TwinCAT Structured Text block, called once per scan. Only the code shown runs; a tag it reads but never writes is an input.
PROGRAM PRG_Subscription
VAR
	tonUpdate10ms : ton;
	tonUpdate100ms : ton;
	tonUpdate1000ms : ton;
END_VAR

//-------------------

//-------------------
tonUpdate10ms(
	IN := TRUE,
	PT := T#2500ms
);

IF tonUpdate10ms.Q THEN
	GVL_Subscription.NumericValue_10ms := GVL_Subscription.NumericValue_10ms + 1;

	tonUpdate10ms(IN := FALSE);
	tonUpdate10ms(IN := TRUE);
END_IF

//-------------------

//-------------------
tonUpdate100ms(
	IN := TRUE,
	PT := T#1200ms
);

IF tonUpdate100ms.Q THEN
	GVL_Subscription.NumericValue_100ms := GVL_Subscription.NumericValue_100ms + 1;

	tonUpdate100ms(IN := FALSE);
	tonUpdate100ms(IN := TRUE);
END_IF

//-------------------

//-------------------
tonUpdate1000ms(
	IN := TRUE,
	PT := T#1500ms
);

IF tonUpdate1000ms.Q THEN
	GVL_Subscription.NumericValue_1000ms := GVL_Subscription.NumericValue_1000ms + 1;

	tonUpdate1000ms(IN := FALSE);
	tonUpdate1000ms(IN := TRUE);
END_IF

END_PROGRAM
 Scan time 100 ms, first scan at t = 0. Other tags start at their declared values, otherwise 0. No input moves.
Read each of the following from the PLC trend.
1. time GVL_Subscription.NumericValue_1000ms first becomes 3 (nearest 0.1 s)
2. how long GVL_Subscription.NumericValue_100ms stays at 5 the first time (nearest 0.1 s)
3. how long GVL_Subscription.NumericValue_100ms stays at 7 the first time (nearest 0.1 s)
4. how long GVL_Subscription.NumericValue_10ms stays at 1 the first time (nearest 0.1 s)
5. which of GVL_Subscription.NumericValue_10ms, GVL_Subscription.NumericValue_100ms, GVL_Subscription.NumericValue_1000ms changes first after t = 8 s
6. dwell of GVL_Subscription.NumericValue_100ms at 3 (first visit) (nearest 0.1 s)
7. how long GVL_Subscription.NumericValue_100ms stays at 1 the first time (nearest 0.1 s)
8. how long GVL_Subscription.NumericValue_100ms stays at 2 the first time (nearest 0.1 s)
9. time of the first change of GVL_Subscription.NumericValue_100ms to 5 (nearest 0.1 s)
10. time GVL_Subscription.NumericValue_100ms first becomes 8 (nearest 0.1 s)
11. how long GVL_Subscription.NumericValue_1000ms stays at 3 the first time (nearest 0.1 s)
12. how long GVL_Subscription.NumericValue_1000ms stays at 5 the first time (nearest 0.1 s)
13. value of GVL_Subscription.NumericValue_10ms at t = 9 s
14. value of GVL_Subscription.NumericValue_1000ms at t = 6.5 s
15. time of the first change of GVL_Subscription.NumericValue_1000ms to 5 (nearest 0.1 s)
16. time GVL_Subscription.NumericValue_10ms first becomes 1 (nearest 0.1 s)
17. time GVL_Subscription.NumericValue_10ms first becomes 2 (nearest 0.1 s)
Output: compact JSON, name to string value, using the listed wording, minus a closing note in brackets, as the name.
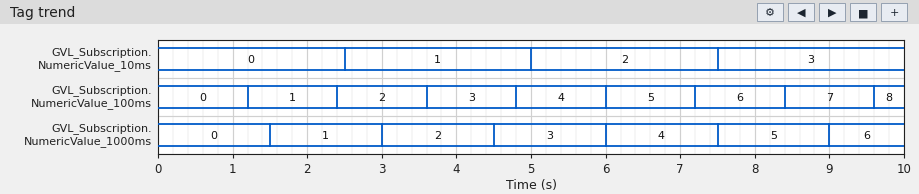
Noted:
{"time GVL_Subscription.NumericValue_1000ms first becomes 3": "4.5 s", "how long GVL_Subscription.NumericValue_100ms stays at 5 the first time": "1.2 s", "how long GVL_Subscription.NumericValue_100ms stays at 7 the first time": "1.2 s", "how long GVL_Subscription.NumericValue_10ms stays at 1 the first time": "2.5 s", "which of GVL_Subscription.NumericValue_10ms, GVL_Subscription.NumericValue_100ms, GVL_Subscription.NumericValue_1000ms changes first after t = 8 s": "GVL_Subscription.NumericValue_100ms", "dwell of GVL_Subscription.NumericValue_100ms at 3 (first visit)": "1.2 s", "how long GVL_Subscription.NumericValue_100ms stays at 1 the first time": "1.2 s", "how long GVL_Subscription.NumericValue_100ms stays at 2 the first time": "1.2 s", "time of the first change of GVL_Subscription.NumericValue_100ms to 5": "6.0 s", "time GVL_Subscription.NumericValue_100ms first becomes 8": "9.6 s", "how long GVL_Subscription.NumericValue_1000ms stays at 3 the first time": "1.5 s", "how long GVL_Subscription.NumericValue_1000ms stays at 5 the first time": "1.5 s", "value of GVL_Subscription.NumericValue_10ms at t = 9 s": "3", "value of GVL_Subscription.NumericValue_1000ms at t = 6.5 s": "4", "time of the first change of GVL_Subscription.NumericValue_1000ms to 5": "7.5 s", "time GVL_Subscription.NumericValue_10ms first becomes 1": "2.5 s", "time GVL_Subscription.NumericValue_10ms first becomes 2": "5.0 s"}
